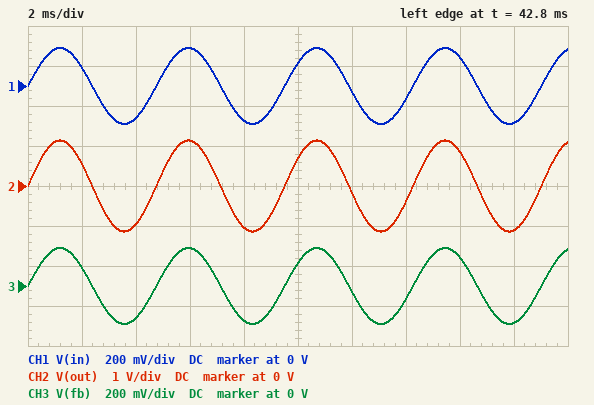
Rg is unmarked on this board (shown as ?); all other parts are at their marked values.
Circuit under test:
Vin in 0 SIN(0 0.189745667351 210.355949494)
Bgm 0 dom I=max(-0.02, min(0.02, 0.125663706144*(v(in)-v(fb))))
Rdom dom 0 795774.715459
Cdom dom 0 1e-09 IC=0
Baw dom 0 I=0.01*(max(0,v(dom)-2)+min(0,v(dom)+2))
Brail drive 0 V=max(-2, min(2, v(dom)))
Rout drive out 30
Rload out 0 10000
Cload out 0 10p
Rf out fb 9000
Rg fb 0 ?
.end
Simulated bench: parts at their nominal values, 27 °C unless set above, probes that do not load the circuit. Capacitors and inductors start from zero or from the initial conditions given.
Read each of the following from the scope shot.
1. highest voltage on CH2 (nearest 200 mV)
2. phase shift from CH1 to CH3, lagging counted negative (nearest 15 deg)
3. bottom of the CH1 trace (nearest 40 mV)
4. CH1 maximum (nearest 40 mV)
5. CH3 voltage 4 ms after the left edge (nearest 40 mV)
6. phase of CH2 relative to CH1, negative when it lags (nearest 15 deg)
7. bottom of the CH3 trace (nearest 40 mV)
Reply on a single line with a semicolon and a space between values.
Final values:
1.2 V; 0 deg; -200 mV; 200 mV; -160 mV; 0 deg; -200 mV
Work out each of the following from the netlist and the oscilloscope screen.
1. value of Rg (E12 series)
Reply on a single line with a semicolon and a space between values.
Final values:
1.8 kΩ
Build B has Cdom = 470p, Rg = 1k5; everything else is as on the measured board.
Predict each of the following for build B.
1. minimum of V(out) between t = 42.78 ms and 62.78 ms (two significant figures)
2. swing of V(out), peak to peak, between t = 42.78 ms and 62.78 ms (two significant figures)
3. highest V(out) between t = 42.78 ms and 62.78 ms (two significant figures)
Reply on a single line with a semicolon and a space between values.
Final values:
-1.3 V; 2.7 V; 1.3 V
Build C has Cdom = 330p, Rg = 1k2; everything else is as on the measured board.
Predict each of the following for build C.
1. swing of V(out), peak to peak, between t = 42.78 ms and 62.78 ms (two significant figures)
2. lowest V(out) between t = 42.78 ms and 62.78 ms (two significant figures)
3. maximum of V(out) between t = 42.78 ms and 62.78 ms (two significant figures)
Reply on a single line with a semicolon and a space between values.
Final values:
3.2 V; -1.6 V; 1.6 V
